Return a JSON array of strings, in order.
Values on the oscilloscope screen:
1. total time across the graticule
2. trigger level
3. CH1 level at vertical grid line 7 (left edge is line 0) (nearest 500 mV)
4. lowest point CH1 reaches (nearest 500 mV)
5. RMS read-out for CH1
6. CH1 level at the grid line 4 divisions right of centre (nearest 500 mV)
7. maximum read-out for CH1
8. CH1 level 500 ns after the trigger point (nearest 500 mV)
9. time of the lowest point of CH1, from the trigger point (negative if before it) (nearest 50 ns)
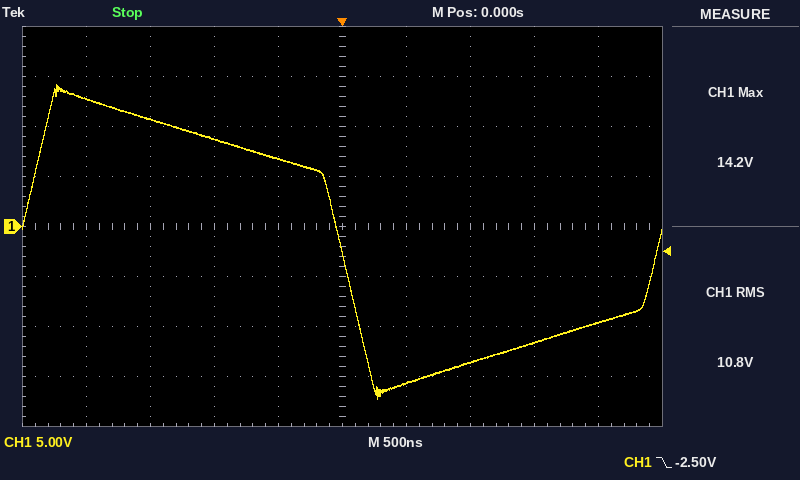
["5 µs", "-2.50 V", "-13.5 V", "-17.5 V", "10.8 V", "-9.5 V", "14.2 V", "-15.5 V", "+300 ns"]
